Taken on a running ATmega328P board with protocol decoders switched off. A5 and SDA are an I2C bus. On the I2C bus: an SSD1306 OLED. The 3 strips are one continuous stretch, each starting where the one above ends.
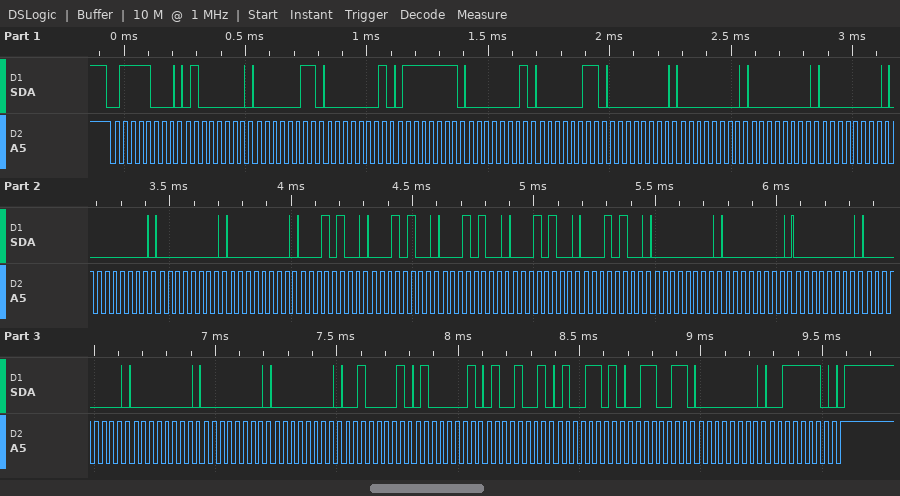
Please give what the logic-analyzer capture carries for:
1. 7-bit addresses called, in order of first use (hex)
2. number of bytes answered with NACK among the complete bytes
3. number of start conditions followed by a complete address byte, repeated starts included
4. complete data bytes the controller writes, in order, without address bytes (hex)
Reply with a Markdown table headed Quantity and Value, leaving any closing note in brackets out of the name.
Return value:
| Quantity | Value |
|---|---|
| 7-bit addresses called, in order of first use | 0x3C |
| number of bytes answered with NACK among the complete bytes | 0 |
| number of start conditions followed by a complete address byte, repeated starts included | 1 |
| complete data bytes the controller writes, in order, without address bytes | 40 03 01 7F 01 03 00 00 00 00 00 00 00 14 14 14 14 14 00 00 00 00 00 00 00 21 41 49 4D 33 00 3E |
